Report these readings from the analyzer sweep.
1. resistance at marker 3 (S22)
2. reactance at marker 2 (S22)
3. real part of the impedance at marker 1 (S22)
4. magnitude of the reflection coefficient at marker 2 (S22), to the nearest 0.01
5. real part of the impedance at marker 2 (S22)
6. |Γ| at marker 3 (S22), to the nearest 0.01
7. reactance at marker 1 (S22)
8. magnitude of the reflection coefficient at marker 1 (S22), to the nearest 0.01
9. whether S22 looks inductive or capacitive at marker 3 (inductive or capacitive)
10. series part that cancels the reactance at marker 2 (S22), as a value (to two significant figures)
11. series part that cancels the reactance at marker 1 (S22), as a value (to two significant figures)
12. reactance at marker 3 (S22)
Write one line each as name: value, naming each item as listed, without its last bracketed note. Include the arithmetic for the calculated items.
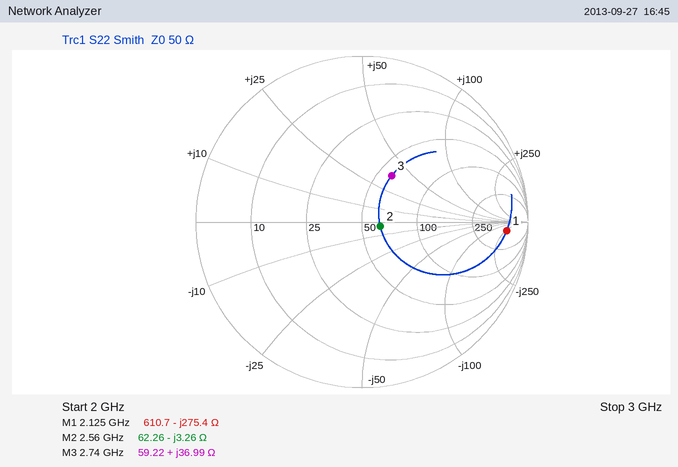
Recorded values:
resistance at marker 3: 59.22 Ω
reactance at marker 2: -3.26 Ω
real part of the impedance at marker 1: 610.7 Ω
magnitude of the reflection coefficient at marker 2 (S22), to the nearest 0.01: 0.11
real part of the impedance at marker 2: 62.26 Ω
|Γ| at marker 3 (S22), to the nearest 0.01: 0.33
reactance at marker 1: -275.4 Ω
magnitude of the reflection coefficient at marker 1 (S22), to the nearest 0.01: 0.87
whether S22 looks inductive or capacitive at marker 3: inductive
series part that cancels the reactance at marker 2 (S22), as a value: L = 3.26 Ω/(2π × 2.56 GHz) ≈ 203 pH, so 200 pH to two significant figures
series part that cancels the reactance at marker 1 (S22), as a value: L = 275.4 Ω/(2π × 2.125 GHz) ≈ 21 nH
reactance at marker 3: +36.99 Ω
